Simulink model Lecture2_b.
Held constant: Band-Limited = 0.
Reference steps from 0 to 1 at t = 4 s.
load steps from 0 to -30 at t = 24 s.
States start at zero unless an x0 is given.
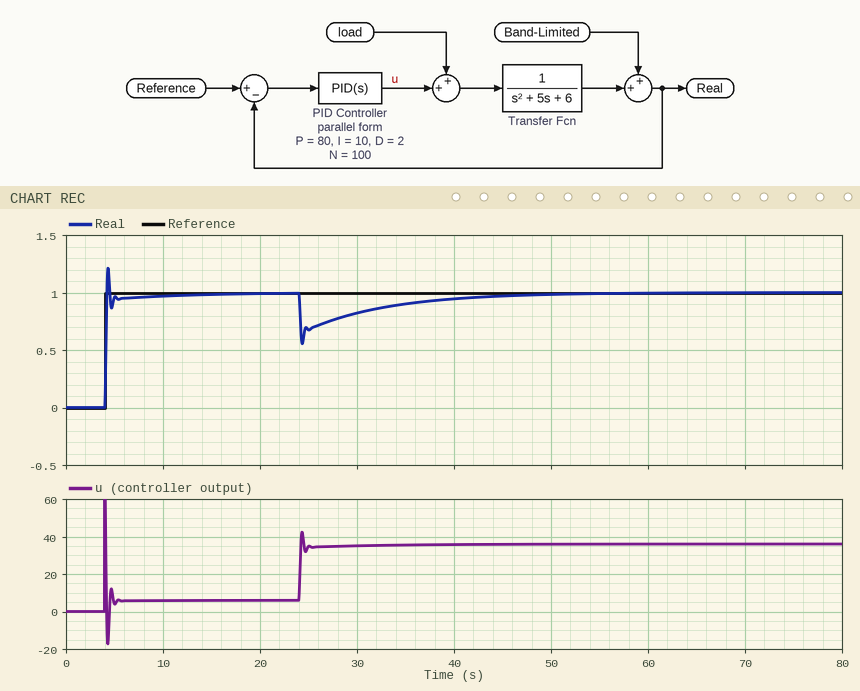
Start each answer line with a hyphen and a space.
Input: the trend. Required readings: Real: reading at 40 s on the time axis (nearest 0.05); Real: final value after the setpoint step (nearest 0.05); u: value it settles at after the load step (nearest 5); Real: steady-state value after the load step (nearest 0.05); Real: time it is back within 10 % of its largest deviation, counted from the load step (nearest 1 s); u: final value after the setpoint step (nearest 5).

- 0.95
- 1.00
- 35
- 1.00
- 18 s
- 5
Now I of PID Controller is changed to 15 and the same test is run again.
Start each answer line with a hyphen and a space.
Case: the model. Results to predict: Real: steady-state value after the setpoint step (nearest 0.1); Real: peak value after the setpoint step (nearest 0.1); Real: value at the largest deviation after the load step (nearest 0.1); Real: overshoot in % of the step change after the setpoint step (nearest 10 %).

- 1.0
- 1.2
- 0.6
- 20 %
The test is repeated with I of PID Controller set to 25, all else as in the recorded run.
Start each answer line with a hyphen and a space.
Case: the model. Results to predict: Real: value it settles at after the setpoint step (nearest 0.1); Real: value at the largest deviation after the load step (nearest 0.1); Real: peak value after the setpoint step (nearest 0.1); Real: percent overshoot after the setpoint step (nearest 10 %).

- 1.0
- 0.6
- 1.2
- 20 %
